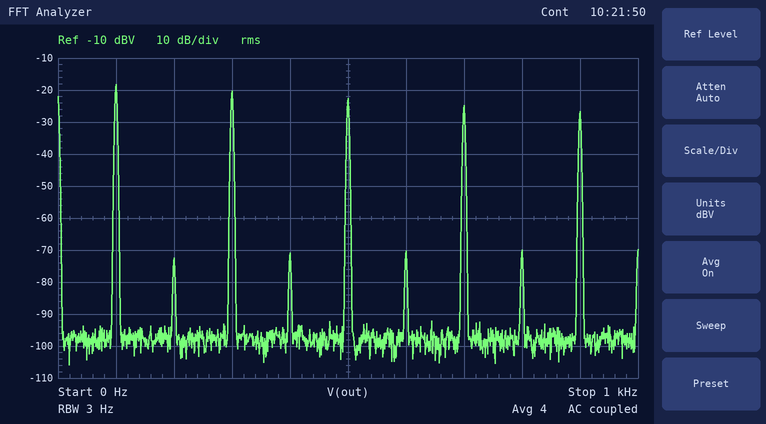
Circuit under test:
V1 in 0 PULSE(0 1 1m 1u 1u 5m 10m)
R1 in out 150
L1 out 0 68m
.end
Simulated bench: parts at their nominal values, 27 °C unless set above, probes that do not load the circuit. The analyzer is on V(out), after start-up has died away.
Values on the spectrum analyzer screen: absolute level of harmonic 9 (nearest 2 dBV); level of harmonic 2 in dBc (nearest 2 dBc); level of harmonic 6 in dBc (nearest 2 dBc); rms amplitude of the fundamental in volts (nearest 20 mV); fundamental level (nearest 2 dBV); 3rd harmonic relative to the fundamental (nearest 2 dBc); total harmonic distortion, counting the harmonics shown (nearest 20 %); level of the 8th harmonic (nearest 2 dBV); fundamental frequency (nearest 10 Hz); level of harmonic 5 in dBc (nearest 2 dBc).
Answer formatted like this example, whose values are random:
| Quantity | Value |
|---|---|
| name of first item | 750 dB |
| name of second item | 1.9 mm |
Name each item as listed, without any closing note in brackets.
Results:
| Quantity | Value |
|---|---|
| absolute level of harmonic 9 | -26 dBV |
| level of harmonic 2 in dBc | -54 dBc |
| level of harmonic 6 in dBc | -52 dBc |
| rms amplitude of the fundamental in volts | 120 mV |
| fundamental level | -18 dBV |
| 3rd harmonic relative to the fundamental | -2 dBc |
| total harmonic distortion, counting the harmonics shown | 120 % |
| level of the 8th harmonic | -70 dBV |
| fundamental frequency | 100 Hz |
| level of harmonic 5 in dBc | -4 dBc |
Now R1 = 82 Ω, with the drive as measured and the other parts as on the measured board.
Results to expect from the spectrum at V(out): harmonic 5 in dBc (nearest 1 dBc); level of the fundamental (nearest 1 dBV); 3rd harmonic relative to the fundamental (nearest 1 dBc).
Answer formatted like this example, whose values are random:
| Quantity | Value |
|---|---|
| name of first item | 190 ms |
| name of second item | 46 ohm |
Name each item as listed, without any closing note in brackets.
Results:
| Quantity | Value |
|---|---|
| harmonic 5 in dBc | -8 dBc |
| level of the fundamental | -14 dBV |
| 3rd harmonic relative to the fundamental | -4 dBc |
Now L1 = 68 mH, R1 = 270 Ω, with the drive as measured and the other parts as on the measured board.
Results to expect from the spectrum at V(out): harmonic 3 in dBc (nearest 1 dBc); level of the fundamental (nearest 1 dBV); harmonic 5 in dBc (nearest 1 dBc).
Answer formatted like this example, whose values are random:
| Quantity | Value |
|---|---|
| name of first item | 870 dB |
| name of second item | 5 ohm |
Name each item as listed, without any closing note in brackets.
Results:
| Quantity | Value |
|---|---|
| harmonic 3 in dBc | -1 dBc |
| level of the fundamental | -23 dBV |
| harmonic 5 in dBc | -2 dBc |
